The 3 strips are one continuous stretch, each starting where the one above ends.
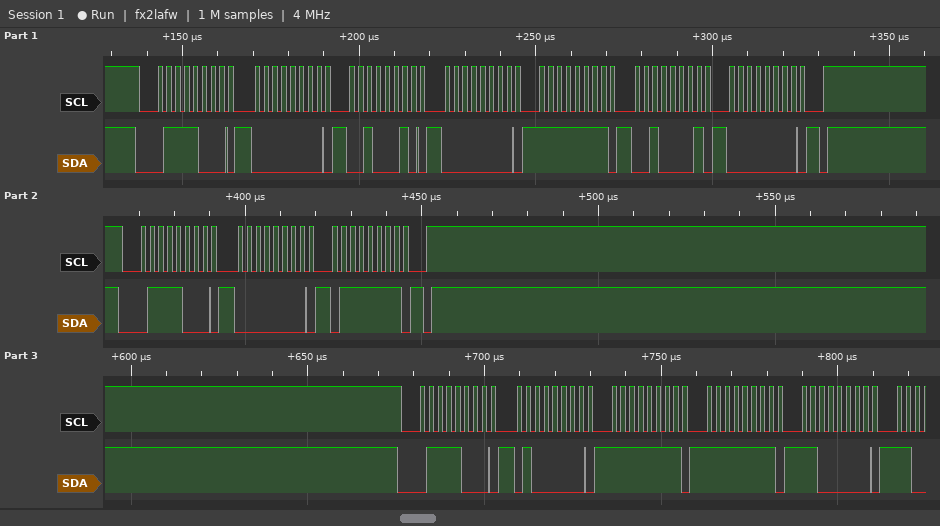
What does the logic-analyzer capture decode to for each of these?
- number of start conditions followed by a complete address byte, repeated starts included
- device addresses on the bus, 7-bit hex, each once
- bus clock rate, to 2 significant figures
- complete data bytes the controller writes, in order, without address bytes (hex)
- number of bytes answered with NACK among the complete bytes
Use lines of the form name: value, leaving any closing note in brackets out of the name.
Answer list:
number of start conditions followed by a complete address byte, repeated starts included: 3
device addresses on the bus, 7-bit hex, each once: 0x3C
bus clock rate, to 2 significant figures: 400 kHz
complete data bytes the controller writes, in order, without address bytes: 00 22 00 FF 21 00 00 7F 40 FF FF C0
number of bytes answered with NACK among the complete bytes: 0
